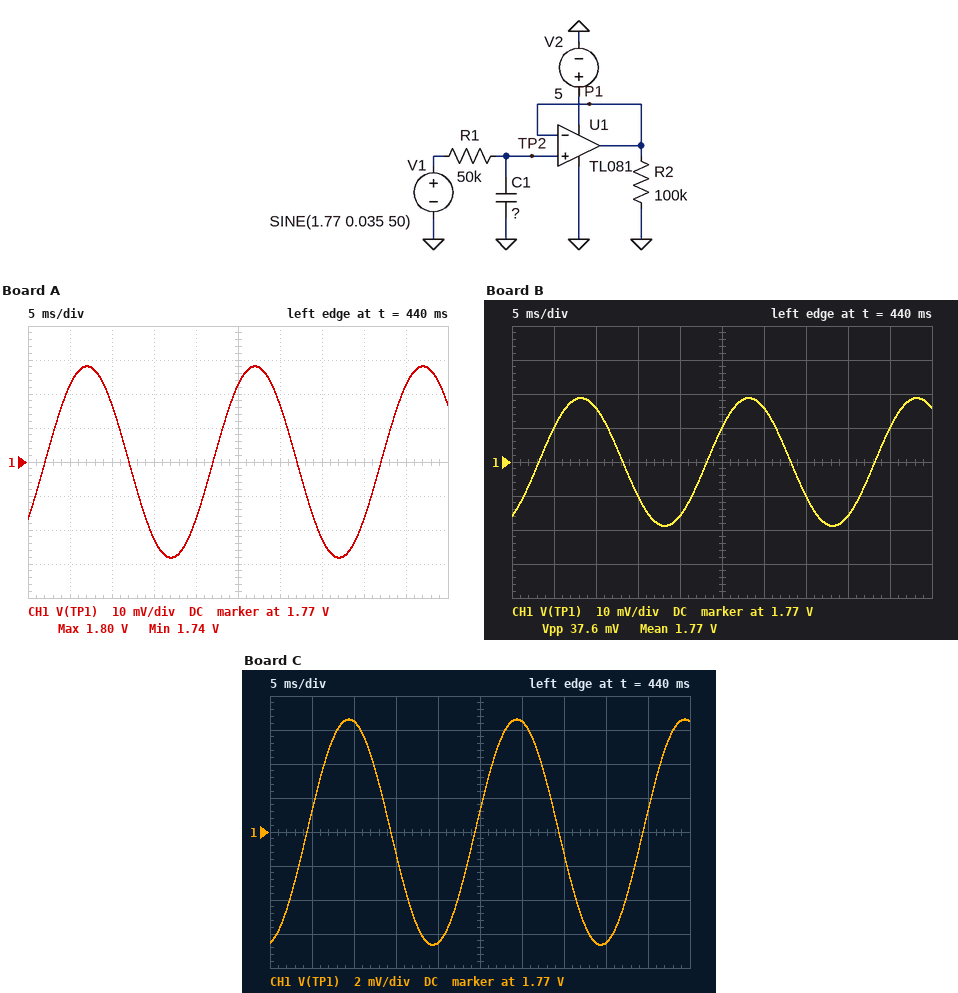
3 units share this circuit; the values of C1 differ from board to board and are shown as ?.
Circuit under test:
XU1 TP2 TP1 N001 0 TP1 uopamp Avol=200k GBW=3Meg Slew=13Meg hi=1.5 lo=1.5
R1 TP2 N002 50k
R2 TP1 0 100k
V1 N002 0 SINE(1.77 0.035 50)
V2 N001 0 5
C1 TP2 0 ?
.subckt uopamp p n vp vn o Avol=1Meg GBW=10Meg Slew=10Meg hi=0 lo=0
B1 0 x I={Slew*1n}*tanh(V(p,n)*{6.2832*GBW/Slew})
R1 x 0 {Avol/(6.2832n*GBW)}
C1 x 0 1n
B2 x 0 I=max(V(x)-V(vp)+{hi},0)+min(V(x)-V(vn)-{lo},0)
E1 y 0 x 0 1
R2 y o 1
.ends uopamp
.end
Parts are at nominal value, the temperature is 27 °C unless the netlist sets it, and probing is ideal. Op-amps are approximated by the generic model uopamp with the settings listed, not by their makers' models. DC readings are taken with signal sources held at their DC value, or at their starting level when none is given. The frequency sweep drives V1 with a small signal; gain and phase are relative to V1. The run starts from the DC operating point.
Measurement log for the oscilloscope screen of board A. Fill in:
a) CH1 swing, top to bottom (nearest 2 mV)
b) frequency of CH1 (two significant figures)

56 mV
50 Hz
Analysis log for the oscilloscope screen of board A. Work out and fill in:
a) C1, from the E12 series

47 nF
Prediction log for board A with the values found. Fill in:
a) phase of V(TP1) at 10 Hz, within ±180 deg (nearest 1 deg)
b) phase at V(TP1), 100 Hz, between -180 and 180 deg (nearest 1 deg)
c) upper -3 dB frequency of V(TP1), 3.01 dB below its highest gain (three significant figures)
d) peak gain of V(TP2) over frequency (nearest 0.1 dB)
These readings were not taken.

-8 deg
-56 deg
67.7 Hz
0 dB
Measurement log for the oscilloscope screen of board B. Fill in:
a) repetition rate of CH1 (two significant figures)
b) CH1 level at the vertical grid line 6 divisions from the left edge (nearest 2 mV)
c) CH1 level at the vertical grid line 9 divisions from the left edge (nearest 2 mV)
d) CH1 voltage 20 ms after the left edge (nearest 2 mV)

50 Hz
1.786 V
1.780 V
1.754 V
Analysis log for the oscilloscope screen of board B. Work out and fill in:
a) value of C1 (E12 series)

100 nF
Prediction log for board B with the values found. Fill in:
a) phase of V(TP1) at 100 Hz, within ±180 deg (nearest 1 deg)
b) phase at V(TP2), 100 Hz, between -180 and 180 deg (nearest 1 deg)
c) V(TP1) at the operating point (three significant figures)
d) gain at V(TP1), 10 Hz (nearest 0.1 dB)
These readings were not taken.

-72 deg
-72 deg
1.77 V
-0.4 dB
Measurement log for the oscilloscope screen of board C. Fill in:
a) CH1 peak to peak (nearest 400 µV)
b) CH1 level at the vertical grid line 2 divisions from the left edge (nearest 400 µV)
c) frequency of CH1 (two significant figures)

13.2 mV
1.7764 V
50 Hz
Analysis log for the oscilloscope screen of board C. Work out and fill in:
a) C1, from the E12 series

330 nF
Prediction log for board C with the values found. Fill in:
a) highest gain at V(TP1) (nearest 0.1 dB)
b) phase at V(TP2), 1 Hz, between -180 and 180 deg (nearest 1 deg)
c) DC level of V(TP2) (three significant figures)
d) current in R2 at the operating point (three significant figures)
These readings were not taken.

0 dB
-6 deg
1.77 V
17.7 µA
